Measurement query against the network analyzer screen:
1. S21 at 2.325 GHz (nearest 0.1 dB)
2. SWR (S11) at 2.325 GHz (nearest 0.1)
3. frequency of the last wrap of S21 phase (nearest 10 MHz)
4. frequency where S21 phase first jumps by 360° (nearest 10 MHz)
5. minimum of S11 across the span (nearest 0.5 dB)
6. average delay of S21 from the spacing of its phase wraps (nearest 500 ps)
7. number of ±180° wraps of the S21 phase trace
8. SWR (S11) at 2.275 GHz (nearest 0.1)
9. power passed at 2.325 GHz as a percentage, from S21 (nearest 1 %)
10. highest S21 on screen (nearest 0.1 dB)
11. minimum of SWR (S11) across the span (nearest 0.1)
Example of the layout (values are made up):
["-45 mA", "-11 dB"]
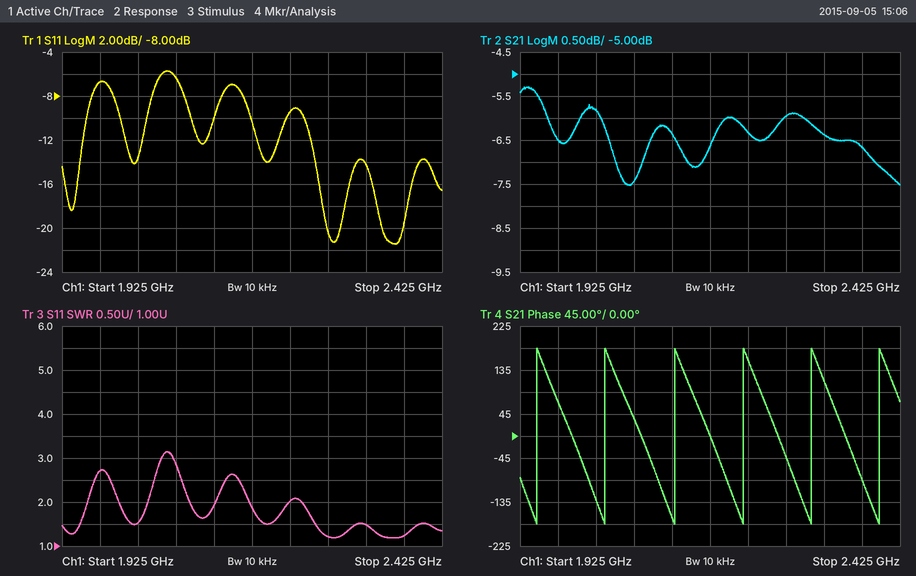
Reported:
["-6.4 dB", "1.5", "2.40 GHz", "1.95 GHz", "-21.5 dB", "11.0 ns", "6", "1.2", "23 %", "-5.3 dB", "1.2"]
